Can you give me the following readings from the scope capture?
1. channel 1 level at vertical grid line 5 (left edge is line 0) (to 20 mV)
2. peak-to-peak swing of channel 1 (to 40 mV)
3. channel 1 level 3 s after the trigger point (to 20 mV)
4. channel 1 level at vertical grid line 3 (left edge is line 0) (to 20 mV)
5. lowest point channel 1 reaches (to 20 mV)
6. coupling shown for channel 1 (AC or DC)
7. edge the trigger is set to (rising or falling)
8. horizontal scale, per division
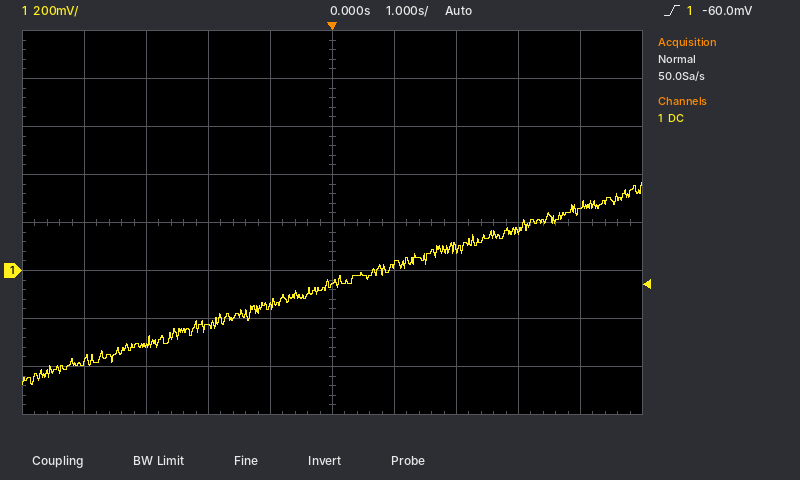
-60 mV
840 mV
160 mV
-240 mV
-480 mV
DC
rising
1 s
